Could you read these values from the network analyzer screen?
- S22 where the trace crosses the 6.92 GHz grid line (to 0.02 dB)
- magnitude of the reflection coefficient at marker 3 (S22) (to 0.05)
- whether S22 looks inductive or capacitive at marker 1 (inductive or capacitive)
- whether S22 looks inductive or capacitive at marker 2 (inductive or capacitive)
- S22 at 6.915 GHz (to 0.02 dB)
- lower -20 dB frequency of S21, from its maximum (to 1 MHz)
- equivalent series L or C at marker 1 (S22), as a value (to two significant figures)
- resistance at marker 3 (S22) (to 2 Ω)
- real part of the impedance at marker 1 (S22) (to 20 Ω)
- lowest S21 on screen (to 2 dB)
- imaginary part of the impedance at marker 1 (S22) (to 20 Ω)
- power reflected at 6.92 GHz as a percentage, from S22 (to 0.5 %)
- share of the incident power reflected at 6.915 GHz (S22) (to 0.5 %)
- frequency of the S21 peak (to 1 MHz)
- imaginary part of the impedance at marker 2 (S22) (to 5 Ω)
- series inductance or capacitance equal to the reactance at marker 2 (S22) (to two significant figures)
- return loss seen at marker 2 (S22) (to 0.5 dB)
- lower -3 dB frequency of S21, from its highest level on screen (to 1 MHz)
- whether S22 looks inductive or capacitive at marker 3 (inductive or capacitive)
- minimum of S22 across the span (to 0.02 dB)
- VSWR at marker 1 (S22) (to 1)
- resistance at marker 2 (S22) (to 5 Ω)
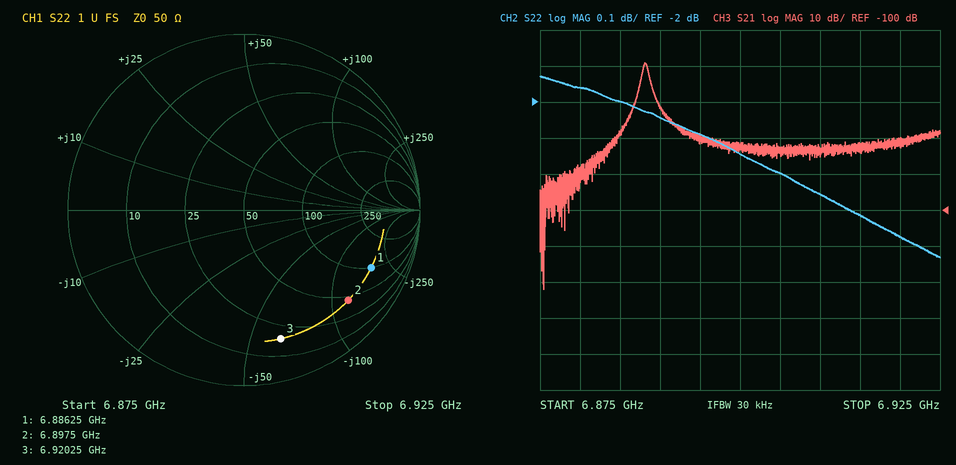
-2.38 dB
0.75
capacitive
capacitive
-2.32 dB
6.885 GHz
130 fF
18 Ω
100 Ω
-122 dB
-180 Ω
58.0 %
58.5 %
6.888 GHz
-120 Ω
190 fF
2.0 dB
6.888 GHz
capacitive
-2.44 dB
9
45 Ω
